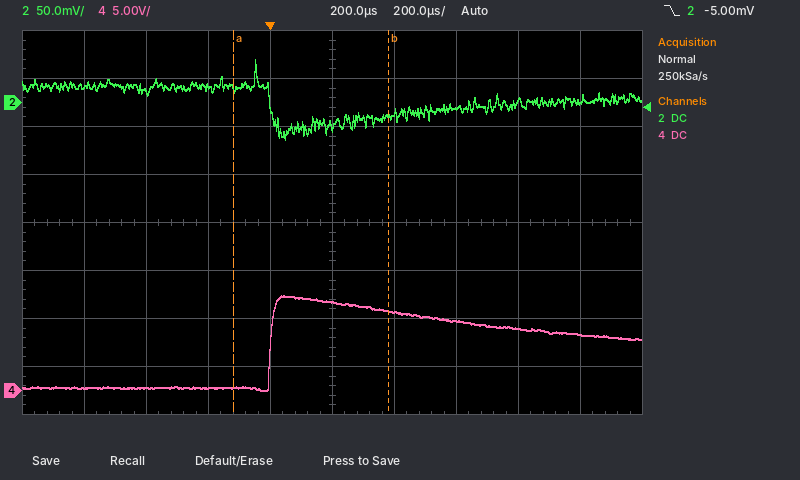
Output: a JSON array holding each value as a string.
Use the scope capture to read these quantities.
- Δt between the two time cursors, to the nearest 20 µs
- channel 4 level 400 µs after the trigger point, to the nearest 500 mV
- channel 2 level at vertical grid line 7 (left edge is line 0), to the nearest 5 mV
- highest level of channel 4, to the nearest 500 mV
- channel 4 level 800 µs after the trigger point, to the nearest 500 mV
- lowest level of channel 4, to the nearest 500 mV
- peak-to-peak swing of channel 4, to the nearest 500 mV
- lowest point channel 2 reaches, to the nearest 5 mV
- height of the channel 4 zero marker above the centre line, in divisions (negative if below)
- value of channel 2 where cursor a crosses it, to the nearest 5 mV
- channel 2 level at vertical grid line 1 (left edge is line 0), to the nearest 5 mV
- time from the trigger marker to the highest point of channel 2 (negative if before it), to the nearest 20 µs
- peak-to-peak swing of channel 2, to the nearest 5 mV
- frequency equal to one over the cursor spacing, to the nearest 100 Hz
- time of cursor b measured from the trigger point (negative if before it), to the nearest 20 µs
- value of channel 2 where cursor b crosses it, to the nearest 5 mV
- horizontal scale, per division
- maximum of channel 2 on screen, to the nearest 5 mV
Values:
["500 µs", "8.0 V", "-5 mV", "10.0 V", "6.5 V", "0.0 V", "10.0 V", "-40 mV", "-3.5 div", "15 mV", "15 mV", "-40 µs", "85 mV", "2.0 kHz", "+380 µs", "-15 mV", "200 µs", "45 mV"]
